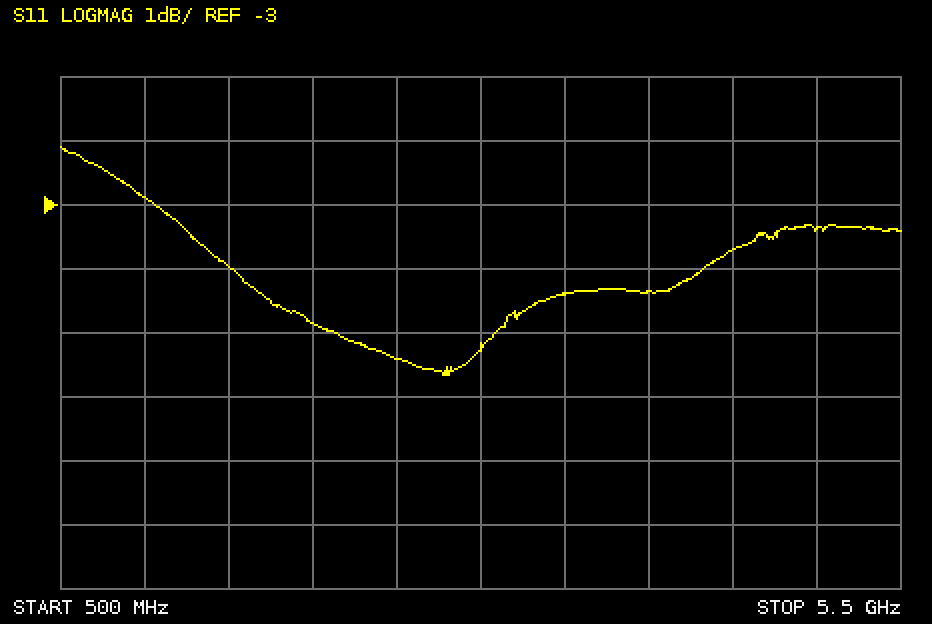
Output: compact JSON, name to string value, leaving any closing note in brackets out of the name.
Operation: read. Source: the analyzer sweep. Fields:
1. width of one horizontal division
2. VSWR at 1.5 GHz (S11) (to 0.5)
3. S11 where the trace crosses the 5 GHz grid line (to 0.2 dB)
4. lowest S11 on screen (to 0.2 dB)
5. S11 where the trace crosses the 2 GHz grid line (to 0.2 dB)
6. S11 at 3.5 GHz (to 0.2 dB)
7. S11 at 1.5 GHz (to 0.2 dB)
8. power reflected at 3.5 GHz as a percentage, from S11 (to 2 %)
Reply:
{"width of one horizontal division": "500 MHz", "VSWR at 1.5 GHz (S11)": "4.5", "S11 where the trace crosses the 5 GHz grid line": "-3.4 dB", "lowest S11 on screen": "-5.6 dB", "S11 where the trace crosses the 2 GHz grid line": "-4.8 dB", "S11 at 3.5 GHz": "-4.4 dB", "S11 at 1.5 GHz": "-4.0 dB", "power reflected at 3.5 GHz as a percentage, from S11": "36 %"}
